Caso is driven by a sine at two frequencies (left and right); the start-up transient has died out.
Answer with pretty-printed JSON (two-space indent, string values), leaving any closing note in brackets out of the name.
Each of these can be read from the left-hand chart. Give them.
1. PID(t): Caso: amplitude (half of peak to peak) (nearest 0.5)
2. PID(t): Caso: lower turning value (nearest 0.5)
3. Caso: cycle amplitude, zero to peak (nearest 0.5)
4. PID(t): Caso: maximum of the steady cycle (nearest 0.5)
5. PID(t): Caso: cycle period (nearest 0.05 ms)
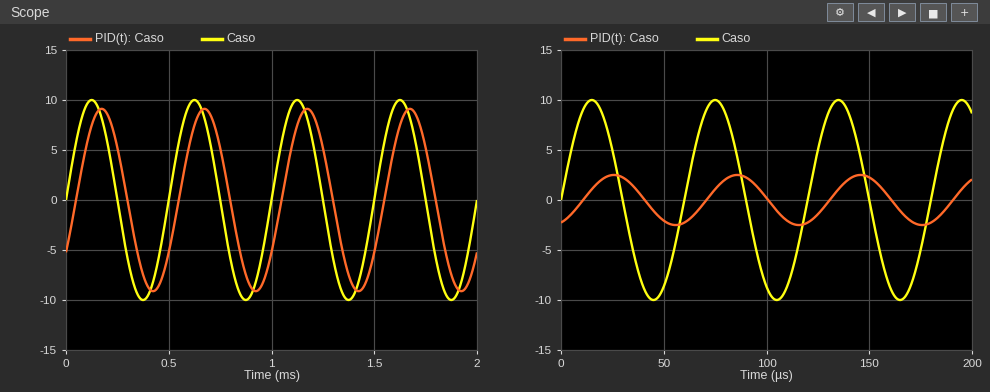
{
  "PID(t): Caso: amplitude (half of peak to peak)": "9.0",
  "PID(t): Caso: lower turning value": "-9.0",
  "Caso: cycle amplitude, zero to peak": "10.0",
  "PID(t): Caso: maximum of the steady cycle": "9.0",
  "PID(t): Caso: cycle period": "0.50 ms"
}
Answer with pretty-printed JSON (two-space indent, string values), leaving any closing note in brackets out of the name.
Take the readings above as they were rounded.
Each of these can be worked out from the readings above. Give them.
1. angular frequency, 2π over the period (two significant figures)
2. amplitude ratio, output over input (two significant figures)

{
  "angular frequency, 2π over the period": "13 rad/ms",
  "amplitude ratio, output over input": "0.90"
}
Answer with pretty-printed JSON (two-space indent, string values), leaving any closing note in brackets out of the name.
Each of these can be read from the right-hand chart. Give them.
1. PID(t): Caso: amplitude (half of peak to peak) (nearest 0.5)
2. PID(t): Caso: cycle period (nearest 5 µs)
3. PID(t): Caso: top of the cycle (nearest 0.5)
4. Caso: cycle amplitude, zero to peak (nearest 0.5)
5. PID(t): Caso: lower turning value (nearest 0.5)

{
  "PID(t): Caso: amplitude (half of peak to peak)": "2.5",
  "PID(t): Caso: cycle period": "60 µs",
  "PID(t): Caso: top of the cycle": "2.5",
  "Caso: cycle amplitude, zero to peak": "10.0",
  "PID(t): Caso: lower turning value": "-2.5"
}
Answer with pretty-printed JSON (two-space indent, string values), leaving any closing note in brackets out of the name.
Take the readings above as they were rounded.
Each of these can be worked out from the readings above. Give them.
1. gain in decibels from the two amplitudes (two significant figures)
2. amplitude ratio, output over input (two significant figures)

{
  "gain in decibels from the two amplitudes": "-12 dB",
  "amplitude ratio, output over input": "0.25"
}
